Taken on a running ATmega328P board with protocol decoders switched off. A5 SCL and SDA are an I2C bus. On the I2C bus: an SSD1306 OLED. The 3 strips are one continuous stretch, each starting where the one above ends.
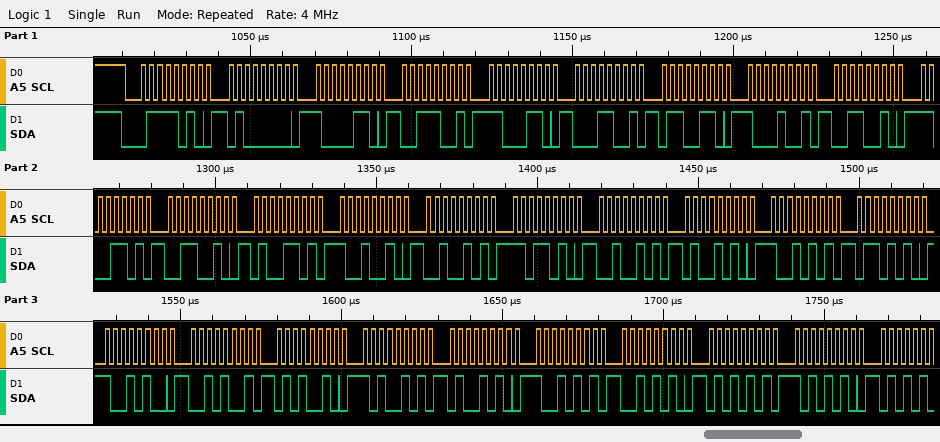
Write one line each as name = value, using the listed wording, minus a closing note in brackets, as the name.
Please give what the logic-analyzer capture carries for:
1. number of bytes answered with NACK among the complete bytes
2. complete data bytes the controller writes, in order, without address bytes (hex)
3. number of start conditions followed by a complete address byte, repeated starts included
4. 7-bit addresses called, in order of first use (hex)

number of bytes answered with NACK among the complete bytes = 0
complete data bytes the controller writes, in order, without address bytes = 40 86 39 C6 19 66 89 32 CD 32 4D 92 25 DA 25 4A 95 6A 94 29 52 A5 4A 95 2A 55 AA
number of start conditions followed by a complete address byte, repeated starts included = 1
7-bit addresses called, in order of first use = 0x3D
